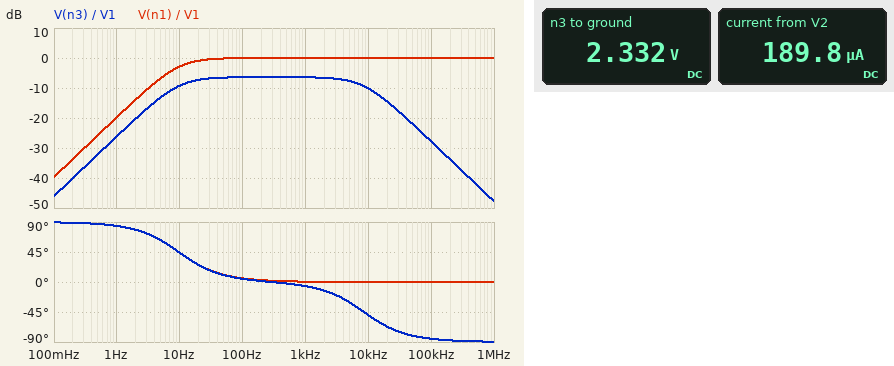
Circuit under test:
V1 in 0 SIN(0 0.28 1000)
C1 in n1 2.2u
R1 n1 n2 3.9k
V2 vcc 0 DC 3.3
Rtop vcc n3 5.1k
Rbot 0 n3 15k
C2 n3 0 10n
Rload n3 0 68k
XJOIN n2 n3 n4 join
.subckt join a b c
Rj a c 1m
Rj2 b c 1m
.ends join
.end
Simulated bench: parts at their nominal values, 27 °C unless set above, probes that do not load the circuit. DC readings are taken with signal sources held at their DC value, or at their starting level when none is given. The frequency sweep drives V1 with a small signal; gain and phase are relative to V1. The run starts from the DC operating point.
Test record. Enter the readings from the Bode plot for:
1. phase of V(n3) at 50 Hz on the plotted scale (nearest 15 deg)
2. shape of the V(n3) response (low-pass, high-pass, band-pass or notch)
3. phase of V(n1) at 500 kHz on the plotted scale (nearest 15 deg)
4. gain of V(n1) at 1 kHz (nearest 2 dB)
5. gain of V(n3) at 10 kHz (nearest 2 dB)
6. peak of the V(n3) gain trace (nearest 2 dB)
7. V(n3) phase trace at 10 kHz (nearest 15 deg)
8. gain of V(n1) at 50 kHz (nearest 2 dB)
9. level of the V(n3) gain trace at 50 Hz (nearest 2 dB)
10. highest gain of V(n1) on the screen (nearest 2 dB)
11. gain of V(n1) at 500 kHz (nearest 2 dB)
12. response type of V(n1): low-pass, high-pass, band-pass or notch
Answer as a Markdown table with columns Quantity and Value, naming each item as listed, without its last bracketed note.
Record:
| Quantity | Value |
|---|---|
| phase of V(n3) at 50 Hz on the plotted scale | 15 deg |
| shape of the V(n3) response | band-pass |
| phase of V(n1) at 500 kHz on the plotted scale | 0 deg |
| gain of V(n1) at 1 kHz | 0 dB |
| gain of V(n3) at 10 kHz | -10 dB |
| peak of the V(n3) gain trace | -6 dB |
| V(n3) phase trace at 10 kHz | -45 deg |
| gain of V(n1) at 50 kHz | 0 dB |
| level of the V(n3) gain trace at 50 Hz | -6 dB |
| highest gain of V(n1) on the screen | 0 dB |
| gain of V(n1) at 500 kHz | 0 dB |
| response type of V(n1): low-pass, high-pass, band-pass or notch | high-pass |
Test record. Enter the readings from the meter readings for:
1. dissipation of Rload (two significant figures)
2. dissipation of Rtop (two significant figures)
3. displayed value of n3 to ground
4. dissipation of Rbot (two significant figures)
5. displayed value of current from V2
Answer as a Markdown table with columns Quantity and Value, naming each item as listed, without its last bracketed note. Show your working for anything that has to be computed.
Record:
| Quantity | Value |
|---|---|
| dissipation of Rload | (2.332 V)^2 / 68 kΩ = 80 µW |
| dissipation of Rtop | (3.3 V - 2.332 V)^2 / 5.1 kΩ = 180 µW |
| displayed value of n3 to ground | 2.332 V |
| dissipation of Rbot | (2.332 V)^2 / 15 kΩ = 360 µW |
| displayed value of current from V2 | 189.8 µA |
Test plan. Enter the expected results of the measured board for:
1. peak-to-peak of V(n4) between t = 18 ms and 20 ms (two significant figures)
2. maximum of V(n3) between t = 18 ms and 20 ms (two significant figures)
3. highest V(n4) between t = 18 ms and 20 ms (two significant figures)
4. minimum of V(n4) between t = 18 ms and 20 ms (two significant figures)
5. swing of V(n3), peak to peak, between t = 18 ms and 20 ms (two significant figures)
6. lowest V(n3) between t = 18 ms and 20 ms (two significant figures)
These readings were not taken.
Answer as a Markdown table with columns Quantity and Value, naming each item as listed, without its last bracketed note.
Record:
| Quantity | Value |
|---|---|
| peak-to-peak of V(n4) between t = 18 ms and 20 ms | 270 mV |
| maximum of V(n3) between t = 18 ms and 20 ms | 2.5 V |
| highest V(n4) between t = 18 ms and 20 ms | 2.5 V |
| minimum of V(n4) between t = 18 ms and 20 ms | 2.2 V |
| swing of V(n3), peak to peak, between t = 18 ms and 20 ms | 270 mV |
| lowest V(n3) between t = 18 ms and 20 ms | 2.2 V |
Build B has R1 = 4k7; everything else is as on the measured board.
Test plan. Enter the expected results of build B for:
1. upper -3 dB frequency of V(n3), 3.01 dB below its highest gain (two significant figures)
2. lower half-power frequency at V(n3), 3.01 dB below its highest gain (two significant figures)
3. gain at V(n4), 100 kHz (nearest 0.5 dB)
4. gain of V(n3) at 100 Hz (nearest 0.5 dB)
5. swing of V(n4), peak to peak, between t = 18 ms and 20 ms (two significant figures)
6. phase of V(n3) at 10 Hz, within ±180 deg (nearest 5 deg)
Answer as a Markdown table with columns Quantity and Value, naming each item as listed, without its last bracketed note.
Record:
| Quantity | Value |
|---|---|
| upper -3 dB frequency of V(n3), 3.01 dB below its highest gain | 7.8 kHz |
| lower half-power frequency at V(n3), 3.01 dB below its highest gain | 8.7 Hz |
| gain at V(n4), 100 kHz | -29.5 dB |
| gain of V(n3) at 100 Hz | -7.5 dB |
| swing of V(n4), peak to peak, between t = 18 ms and 20 ms | 240 mV |
| phase of V(n3) at 10 Hz, within ±180 deg | 40 deg |
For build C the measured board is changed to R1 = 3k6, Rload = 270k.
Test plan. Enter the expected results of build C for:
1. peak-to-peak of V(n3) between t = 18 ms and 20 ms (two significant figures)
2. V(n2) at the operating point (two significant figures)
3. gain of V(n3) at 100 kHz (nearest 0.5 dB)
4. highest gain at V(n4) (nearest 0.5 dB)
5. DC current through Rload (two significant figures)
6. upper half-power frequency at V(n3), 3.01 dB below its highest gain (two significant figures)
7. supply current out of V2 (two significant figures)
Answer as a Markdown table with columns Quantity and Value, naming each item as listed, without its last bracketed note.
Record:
| Quantity | Value |
|---|---|
| peak-to-peak of V(n3) between t = 18 ms and 20 ms | 280 mV |
| V(n2) at the operating point | 2.4 V |
| gain of V(n3) at 100 kHz | -27.0 dB |
| highest gain at V(n4) | -6.0 dB |
| DC current through Rload | 9.0 µA |
| upper half-power frequency at V(n3), 3.01 dB below its highest gain | 8.7 kHz |
| supply current out of V2 | 170 µA |
